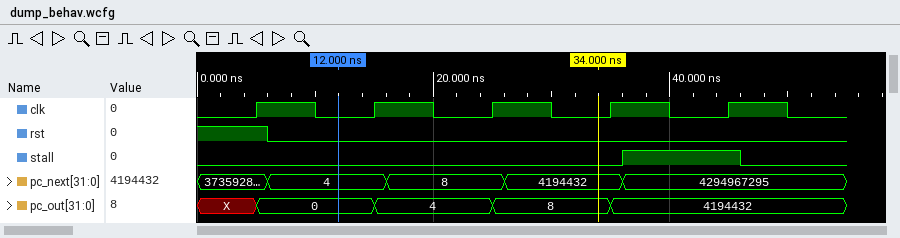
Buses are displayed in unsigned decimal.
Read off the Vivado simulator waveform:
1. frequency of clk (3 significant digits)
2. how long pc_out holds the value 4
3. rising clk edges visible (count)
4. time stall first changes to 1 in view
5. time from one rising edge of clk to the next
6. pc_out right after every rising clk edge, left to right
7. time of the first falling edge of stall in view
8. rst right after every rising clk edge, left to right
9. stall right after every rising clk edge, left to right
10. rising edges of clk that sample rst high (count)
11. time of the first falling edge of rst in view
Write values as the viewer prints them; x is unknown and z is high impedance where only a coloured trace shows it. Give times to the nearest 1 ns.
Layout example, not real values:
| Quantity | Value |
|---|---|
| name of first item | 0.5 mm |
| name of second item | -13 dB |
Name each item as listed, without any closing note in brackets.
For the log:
| Quantity | Value |
|---|---|
| frequency of clk | 100 MHz |
| how long pc_out holds the value 4 | 10 ns |
| rising clk edges visible | 5 |
| time stall first changes to 1 in view | 36 ns |
| time from one rising edge of clk to the next | 10 ns |
| pc_out right after every rising clk edge, left to right | 0, 4, 8, 4194432, 4194432 |
| time of the first falling edge of stall in view | 46 ns |
| rst right after every rising clk edge, left to right | 1 0 0 0 0 |
| stall right after every rising clk edge, left to right | 0 0 0 0 1 |
| rising edges of clk that sample rst high | 1 |
| time of the first falling edge of rst in view | 6 ns |
